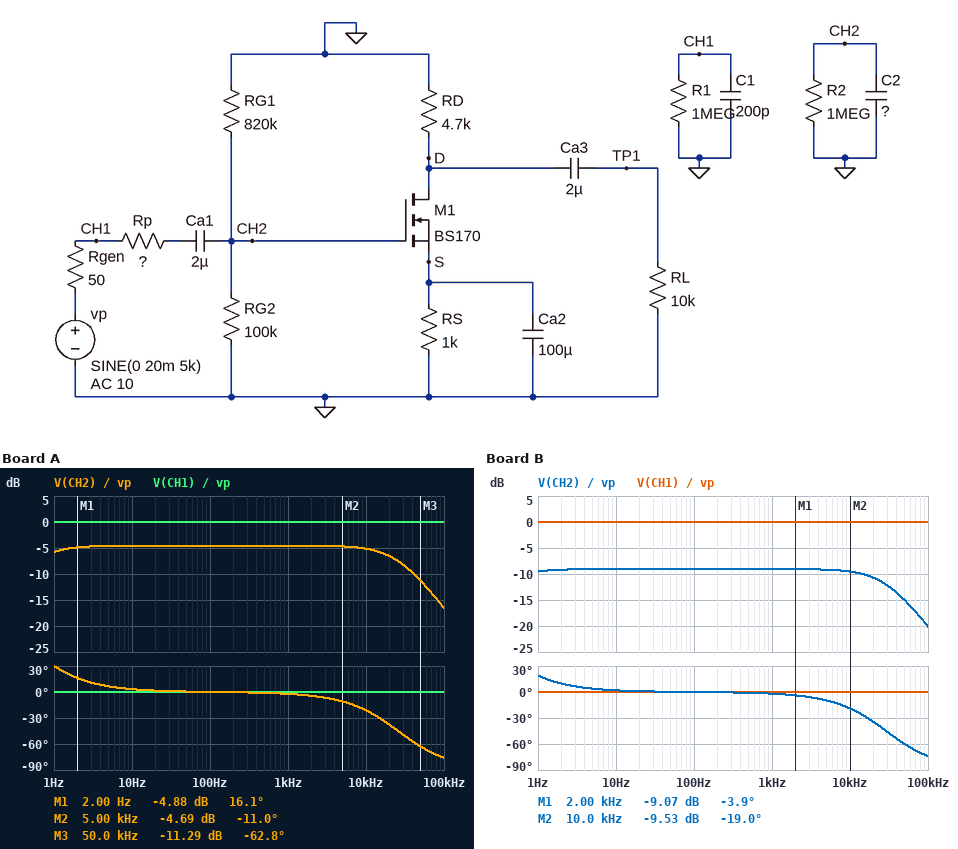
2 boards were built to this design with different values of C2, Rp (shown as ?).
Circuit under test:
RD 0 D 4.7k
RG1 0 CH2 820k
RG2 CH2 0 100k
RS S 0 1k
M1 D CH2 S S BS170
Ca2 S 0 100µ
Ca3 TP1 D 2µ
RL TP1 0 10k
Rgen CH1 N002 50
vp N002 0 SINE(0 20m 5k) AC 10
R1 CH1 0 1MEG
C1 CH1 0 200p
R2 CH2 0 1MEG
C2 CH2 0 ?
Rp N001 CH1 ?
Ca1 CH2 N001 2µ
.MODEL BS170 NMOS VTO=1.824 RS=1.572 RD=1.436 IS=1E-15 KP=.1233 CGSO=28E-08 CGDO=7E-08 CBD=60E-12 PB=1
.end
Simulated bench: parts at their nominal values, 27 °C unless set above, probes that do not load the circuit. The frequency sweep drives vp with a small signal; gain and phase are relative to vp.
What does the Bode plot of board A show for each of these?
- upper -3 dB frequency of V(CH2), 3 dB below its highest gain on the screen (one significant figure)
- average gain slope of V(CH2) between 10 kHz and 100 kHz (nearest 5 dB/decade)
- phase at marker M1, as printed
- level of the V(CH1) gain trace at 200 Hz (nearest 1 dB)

30 kHz
-10 dB/decade
16.1 deg
0 dB
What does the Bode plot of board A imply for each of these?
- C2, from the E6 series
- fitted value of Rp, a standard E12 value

150 pF
56 kΩ
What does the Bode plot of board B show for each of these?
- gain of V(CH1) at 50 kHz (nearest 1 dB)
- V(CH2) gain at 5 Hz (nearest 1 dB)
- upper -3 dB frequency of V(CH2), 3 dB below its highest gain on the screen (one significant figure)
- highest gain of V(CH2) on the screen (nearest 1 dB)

0 dB
-9 dB
30 kHz
-9 dB
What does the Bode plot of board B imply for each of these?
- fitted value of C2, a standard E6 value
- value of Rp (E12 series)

68 pF
150 kΩ
